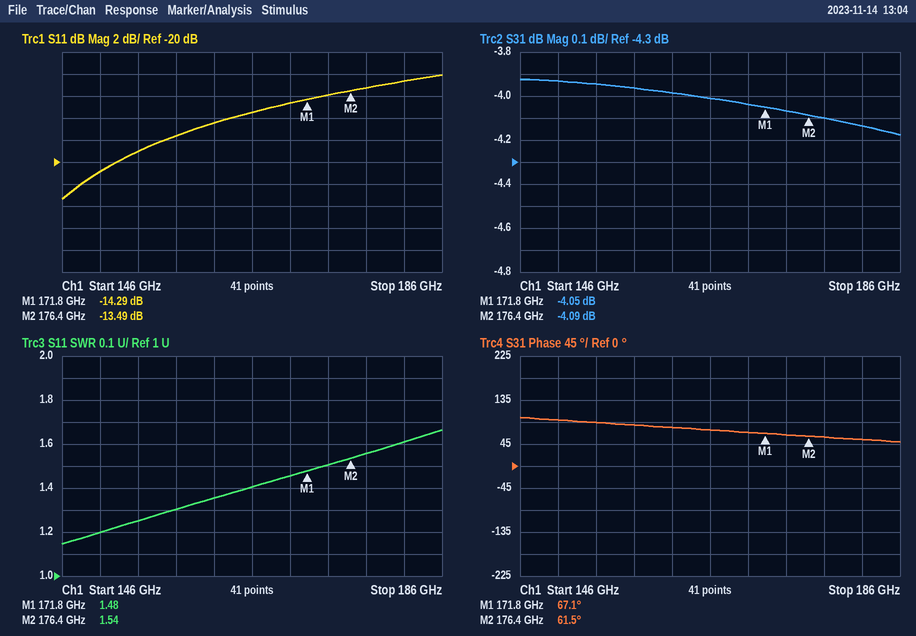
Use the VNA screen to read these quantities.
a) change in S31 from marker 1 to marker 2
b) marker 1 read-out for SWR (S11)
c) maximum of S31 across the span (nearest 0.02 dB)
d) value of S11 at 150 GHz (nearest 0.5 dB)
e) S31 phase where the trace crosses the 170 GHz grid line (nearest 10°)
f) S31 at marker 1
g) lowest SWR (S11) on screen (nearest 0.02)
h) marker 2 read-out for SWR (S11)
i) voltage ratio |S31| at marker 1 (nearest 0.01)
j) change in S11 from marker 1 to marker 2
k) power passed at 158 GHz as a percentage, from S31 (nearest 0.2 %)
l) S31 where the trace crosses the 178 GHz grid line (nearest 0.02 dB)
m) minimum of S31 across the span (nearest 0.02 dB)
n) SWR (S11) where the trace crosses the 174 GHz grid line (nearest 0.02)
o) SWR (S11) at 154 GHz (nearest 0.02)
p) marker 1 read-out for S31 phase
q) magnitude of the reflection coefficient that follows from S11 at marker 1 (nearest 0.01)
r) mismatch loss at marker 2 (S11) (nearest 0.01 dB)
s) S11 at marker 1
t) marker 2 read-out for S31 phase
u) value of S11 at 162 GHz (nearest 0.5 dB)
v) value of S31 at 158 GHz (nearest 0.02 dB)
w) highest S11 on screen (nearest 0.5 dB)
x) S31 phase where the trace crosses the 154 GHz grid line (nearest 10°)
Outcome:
-0.04 dB
1.48
-3.92 dB
-21.0 dB
70°
-4.05 dB
1.14
1.54
0.63
0.80 dB
40.2 %
-4.10 dB
-4.18 dB
1.50
1.26
67.1°
0.19
0.20 dB
-14.29 dB
61.5°
-16.5 dB
-3.96 dB
-12.0 dB
90°
